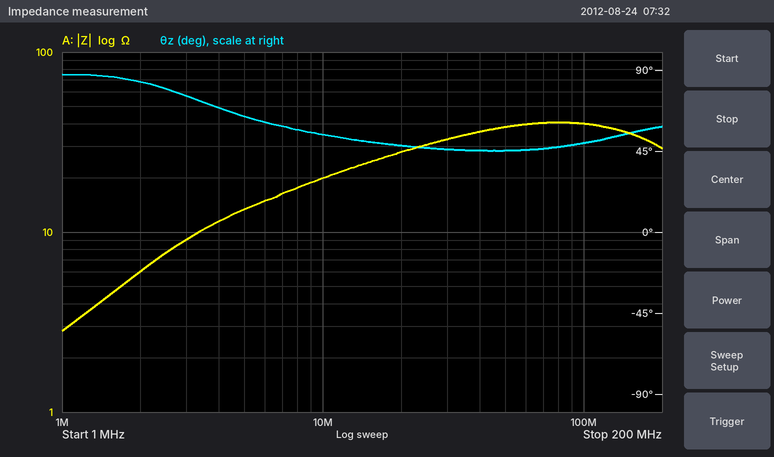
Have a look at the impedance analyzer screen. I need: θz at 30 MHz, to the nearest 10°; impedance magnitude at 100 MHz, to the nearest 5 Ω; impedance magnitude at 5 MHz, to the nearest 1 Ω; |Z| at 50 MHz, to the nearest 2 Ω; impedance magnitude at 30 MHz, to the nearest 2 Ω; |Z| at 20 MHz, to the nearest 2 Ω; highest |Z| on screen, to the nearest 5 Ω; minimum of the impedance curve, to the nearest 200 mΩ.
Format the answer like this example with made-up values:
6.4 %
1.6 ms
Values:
50°
40 Ω
13 Ω
38 Ω
32 Ω
28 Ω
40 Ω
2.8 Ω
